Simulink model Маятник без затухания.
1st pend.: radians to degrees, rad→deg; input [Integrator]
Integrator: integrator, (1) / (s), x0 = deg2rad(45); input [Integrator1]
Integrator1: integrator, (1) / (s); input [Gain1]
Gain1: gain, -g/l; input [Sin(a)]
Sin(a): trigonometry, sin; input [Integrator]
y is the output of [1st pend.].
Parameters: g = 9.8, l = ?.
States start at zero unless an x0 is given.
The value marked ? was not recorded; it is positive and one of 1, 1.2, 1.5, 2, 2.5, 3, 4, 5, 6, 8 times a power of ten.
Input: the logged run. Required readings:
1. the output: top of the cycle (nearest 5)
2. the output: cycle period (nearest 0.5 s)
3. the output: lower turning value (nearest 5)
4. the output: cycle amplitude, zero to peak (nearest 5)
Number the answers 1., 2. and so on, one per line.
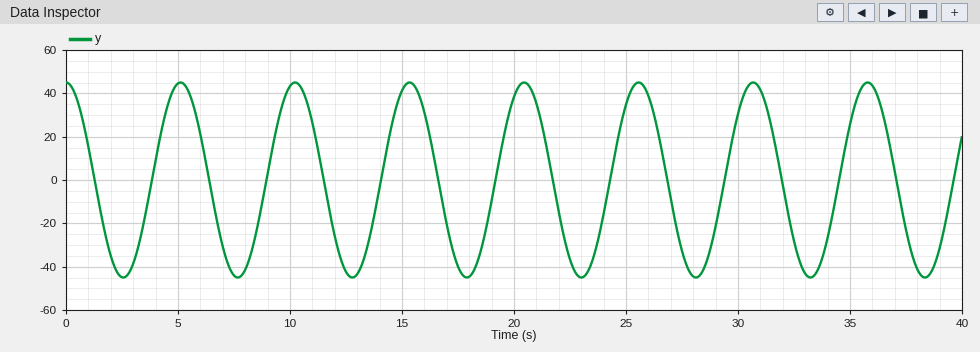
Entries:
1. 45
2. 5.0 s
3. -45
4. 45
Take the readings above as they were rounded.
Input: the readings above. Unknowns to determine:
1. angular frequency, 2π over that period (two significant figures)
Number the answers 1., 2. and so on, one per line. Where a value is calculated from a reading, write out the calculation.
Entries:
1. 2π / 5 = 1.3 rad/s
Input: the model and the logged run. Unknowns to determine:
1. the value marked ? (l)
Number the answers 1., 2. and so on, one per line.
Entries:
1. 6
